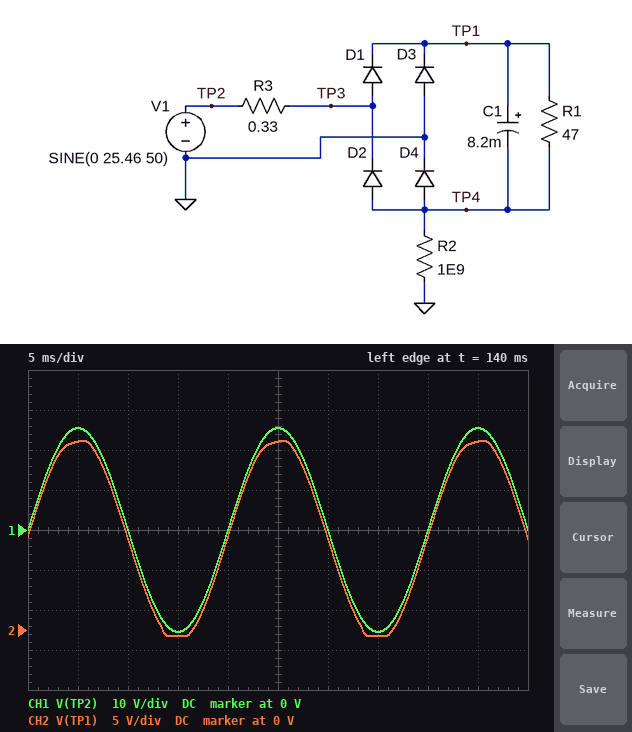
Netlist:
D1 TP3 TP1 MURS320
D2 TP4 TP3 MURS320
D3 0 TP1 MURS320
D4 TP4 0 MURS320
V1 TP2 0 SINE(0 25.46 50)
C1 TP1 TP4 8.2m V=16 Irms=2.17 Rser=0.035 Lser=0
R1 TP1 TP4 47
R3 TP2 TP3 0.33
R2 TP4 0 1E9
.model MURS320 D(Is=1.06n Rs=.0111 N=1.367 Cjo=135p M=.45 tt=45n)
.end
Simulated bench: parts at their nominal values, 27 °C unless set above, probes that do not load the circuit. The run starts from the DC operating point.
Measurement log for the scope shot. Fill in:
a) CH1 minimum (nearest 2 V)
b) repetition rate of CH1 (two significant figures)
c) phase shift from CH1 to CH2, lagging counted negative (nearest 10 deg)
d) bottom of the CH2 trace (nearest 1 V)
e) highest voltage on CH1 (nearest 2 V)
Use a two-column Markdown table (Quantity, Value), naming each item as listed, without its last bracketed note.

| Quantity | Value |
|---|---|
| CH1 minimum | -26 V |
| repetition rate of CH1 | 50 Hz |
| phase shift from CH1 to CH2, lagging counted negative | 0 deg |
| bottom of the CH2 trace | -1 V |
| highest voltage on CH1 | 26 V |
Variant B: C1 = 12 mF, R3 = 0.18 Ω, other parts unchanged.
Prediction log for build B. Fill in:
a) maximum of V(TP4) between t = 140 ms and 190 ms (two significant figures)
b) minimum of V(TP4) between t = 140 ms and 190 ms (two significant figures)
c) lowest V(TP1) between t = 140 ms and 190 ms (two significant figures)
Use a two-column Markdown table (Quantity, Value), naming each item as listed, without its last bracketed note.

| Quantity | Value |
|---|---|
| maximum of V(TP4) between t = 140 ms and 190 ms | 820 mV |
| minimum of V(TP4) between t = 140 ms and 190 ms | -24 V |
| lowest V(TP1) between t = 140 ms and 190 ms | -820 mV |
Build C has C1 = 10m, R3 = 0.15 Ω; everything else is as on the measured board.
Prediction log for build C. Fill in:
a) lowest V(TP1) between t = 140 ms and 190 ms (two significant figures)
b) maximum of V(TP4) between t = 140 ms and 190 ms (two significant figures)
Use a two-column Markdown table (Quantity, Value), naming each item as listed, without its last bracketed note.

| Quantity | Value |
|---|---|
| lowest V(TP1) between t = 140 ms and 190 ms | -830 mV |
| maximum of V(TP4) between t = 140 ms and 190 ms | 830 mV |
